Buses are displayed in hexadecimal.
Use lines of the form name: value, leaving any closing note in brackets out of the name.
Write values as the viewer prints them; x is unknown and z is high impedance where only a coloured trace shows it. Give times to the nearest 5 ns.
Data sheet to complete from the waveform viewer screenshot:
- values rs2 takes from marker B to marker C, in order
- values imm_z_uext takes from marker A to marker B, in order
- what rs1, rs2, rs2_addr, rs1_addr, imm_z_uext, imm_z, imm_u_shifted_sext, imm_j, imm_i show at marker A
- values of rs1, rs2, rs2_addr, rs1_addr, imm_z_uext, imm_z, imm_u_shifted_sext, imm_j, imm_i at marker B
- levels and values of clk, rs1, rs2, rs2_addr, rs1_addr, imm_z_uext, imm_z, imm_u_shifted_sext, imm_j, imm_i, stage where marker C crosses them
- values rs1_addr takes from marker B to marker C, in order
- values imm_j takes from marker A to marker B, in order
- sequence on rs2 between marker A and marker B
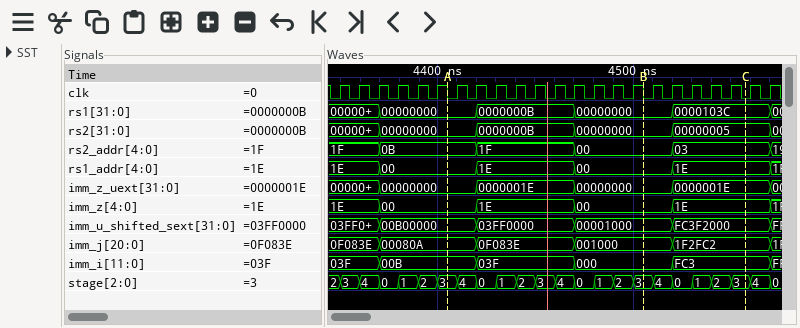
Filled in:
values rs2 takes from marker B to marker C, in order: 00000000, 00000005
values imm_z_uext takes from marker A to marker B, in order: 00000000, 0000001E, 00000000
what rs1, rs2, rs2_addr, rs1_addr, imm_z_uext, imm_z, imm_u_shifted_sext, imm_j, imm_i show at marker A: rs1=00000000, rs2=00000000, rs2_addr=0B, rs1_addr=00, imm_z_uext=00000000, imm_z=00, imm_u_shifted_sext=00B00000, imm_j=00080A, imm_i=00B
values of rs1, rs2, rs2_addr, rs1_addr, imm_z_uext, imm_z, imm_u_shifted_sext, imm_j, imm_i at marker B: rs1=00000000, rs2=00000000, rs2_addr=00, rs1_addr=00, imm_z_uext=00000000, imm_z=00, imm_u_shifted_sext=00001000, imm_j=001000, imm_i=000
levels and values of clk, rs1, rs2, rs2_addr, rs1_addr, imm_z_uext, imm_z, imm_u_shifted_sext, imm_j, imm_i, stage where marker C crosses them: clk=0, rs1=0000103C, rs2=00000005, rs2_addr=03, rs1_addr=1E, imm_z_uext=0000001E, imm_z=1E, imm_u_shifted_sext=FC3F2000, imm_j=1F2FC2, imm_i=FC3, stage=3
values rs1_addr takes from marker B to marker C, in order: 00, 1E
values imm_j takes from marker A to marker B, in order: 00080A, 0F083E, 001000
sequence on rs2 between marker A and marker B: 00000000, 0000000B, 00000000
